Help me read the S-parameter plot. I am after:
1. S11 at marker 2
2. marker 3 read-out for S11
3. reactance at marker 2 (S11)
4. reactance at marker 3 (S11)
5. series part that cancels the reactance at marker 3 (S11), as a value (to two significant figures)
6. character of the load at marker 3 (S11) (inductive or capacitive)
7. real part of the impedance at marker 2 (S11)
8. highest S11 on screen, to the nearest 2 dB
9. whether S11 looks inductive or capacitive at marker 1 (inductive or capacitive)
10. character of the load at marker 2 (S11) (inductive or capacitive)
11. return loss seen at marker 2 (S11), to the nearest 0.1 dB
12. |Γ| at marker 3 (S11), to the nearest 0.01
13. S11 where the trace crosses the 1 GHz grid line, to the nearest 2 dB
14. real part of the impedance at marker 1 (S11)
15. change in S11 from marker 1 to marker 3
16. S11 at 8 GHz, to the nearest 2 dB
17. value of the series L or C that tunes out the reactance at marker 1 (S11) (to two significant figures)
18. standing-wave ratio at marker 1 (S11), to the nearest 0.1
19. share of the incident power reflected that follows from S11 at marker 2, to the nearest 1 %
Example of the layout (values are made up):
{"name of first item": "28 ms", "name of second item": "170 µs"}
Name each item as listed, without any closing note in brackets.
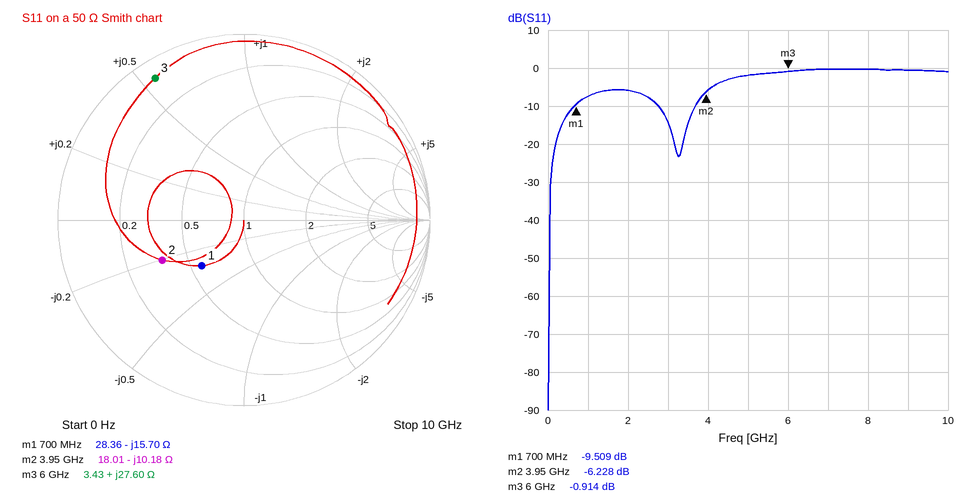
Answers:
{"S11 at marker 2": "-6.228 dB", "marker 3 read-out for S11": "-0.914 dB", "reactance at marker 2": "-10.18 Ω", "reactance at marker 3": "+27.60 Ω", "series part that cancels the reactance at marker 3 (S11), as a value": "960 fF", "character of the load at marker 3 (S11)": "inductive", "real part of the impedance at marker 2": "18.01 Ω", "highest S11 on screen, to the nearest 2 dB": "0 dB", "whether S11 looks inductive or capacitive at marker 1": "capacitive", "character of the load at marker 2 (S11)": "capacitive", "return loss seen at marker 2 (S11), to the nearest 0.1 dB": "6.2 dB", "|Γ| at marker 3 (S11), to the nearest 0.01": "0.90", "S11 where the trace crosses the 1 GHz grid line, to the nearest 2 dB": "-8 dB", "real part of the impedance at marker 1": "28.36 Ω", "change in S11 from marker 1 to marker 3": "8.595 dB", "S11 at 8 GHz, to the nearest 2 dB": "0 dB", "value of the series L or C that tunes out the reactance at marker 1 (S11)": "3.6 nH", "standing-wave ratio at marker 1 (S11), to the nearest 0.1": "2.0", "share of the incident power reflected that follows from S11 at marker 2, to the nearest 1 %": "24 %"}
